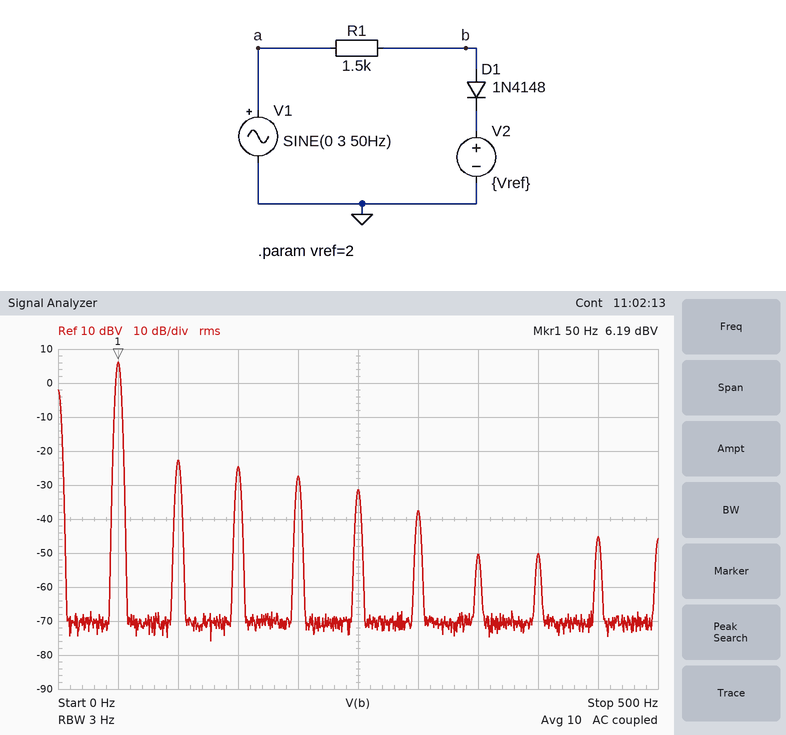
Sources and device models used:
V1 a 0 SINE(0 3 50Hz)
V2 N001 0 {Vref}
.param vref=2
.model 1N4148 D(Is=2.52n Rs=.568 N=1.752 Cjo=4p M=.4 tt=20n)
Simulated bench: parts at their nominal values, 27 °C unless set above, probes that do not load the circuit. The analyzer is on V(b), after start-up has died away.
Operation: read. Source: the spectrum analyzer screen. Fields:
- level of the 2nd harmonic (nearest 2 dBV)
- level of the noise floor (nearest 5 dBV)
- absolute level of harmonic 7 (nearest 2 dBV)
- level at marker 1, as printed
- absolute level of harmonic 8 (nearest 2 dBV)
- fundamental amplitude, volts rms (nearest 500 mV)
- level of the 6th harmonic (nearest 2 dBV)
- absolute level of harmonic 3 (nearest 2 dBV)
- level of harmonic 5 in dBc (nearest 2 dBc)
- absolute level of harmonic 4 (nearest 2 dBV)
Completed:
-22 dBV
-70 dBV
-50 dBV
6.19 dBV
-50 dBV
2.0 V
-38 dBV
-24 dBV
-38 dBc
-28 dBV
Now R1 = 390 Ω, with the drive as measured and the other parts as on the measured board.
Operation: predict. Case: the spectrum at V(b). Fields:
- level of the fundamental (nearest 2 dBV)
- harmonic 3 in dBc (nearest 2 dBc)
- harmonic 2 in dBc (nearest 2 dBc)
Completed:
6 dBV
-32 dBc
-30 dBc
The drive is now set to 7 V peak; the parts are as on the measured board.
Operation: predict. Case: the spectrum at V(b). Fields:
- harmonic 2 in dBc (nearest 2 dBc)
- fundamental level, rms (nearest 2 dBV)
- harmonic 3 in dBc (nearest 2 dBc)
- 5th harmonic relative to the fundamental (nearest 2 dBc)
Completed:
-12 dBc
12 dBV
-22 dBc
-30 dBc
